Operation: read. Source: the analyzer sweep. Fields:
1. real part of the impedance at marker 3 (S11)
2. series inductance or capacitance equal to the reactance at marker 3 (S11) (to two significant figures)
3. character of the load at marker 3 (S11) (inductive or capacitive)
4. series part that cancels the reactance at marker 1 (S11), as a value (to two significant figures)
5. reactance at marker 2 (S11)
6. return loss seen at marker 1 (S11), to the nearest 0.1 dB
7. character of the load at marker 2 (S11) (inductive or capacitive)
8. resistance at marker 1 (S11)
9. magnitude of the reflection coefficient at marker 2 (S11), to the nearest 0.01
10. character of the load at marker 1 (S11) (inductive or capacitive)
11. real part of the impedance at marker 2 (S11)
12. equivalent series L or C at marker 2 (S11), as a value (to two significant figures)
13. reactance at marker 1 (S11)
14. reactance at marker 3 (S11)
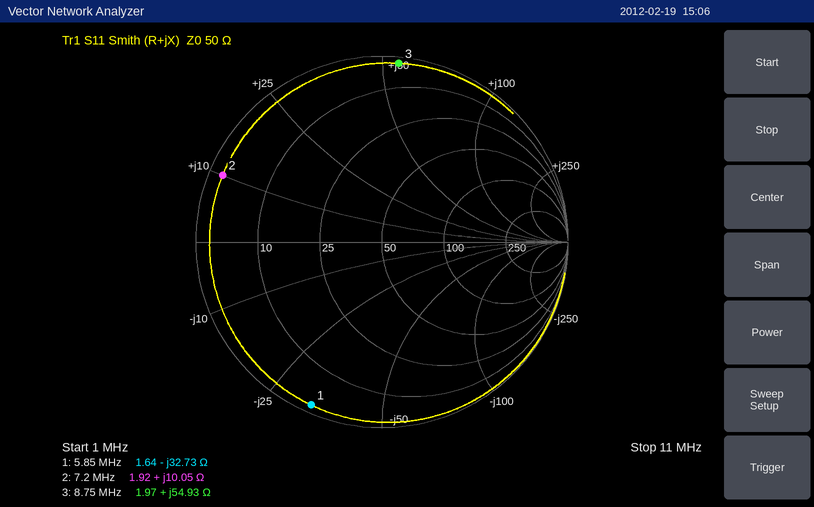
1.97 Ω
1.00 µH
inductive
890 nH
+10.05 Ω
0.4 dB
inductive
1.64 Ω
0.93
capacitive
1.92 Ω
220 nH
-32.73 Ω
+54.93 Ω
